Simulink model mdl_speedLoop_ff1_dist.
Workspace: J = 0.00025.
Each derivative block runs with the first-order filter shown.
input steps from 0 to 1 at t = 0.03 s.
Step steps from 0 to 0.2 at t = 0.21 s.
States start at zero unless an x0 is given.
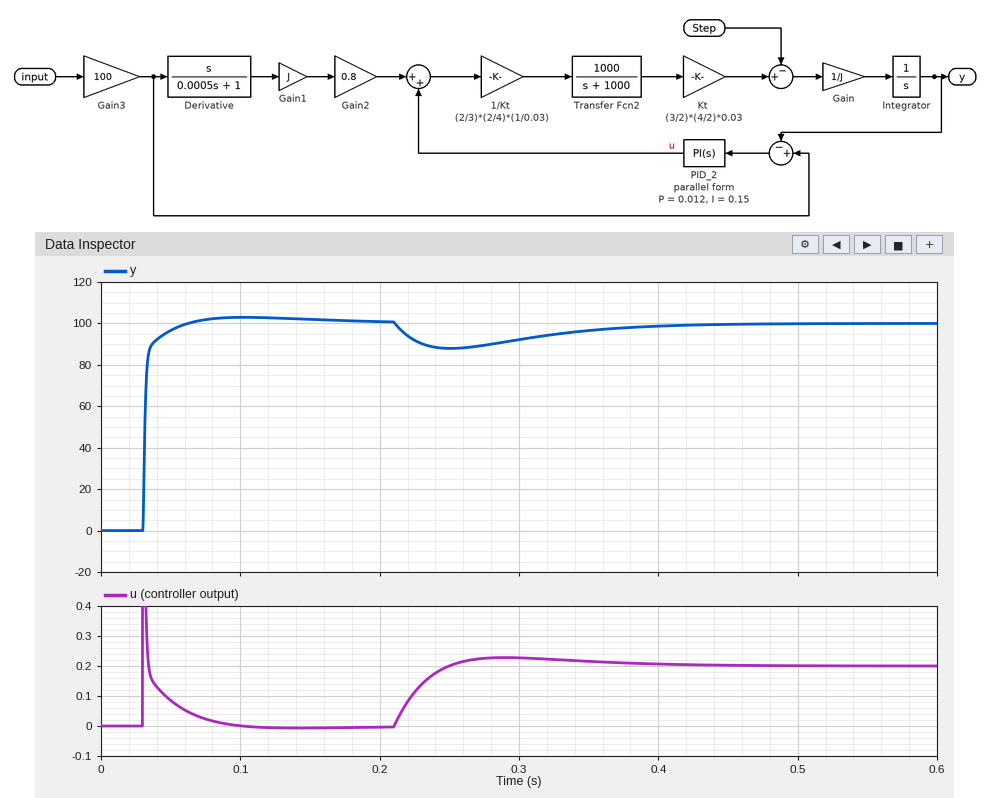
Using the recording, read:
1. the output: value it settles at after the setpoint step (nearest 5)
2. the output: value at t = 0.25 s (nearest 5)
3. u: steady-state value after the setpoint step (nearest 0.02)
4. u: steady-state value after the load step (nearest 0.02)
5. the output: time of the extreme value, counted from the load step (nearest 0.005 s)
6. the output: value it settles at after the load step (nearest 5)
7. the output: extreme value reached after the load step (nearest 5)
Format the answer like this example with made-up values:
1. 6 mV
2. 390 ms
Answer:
1. 100
2. 90
3. 0.00
4. 0.20
5. 0.040 s
6. 100
7. 90
